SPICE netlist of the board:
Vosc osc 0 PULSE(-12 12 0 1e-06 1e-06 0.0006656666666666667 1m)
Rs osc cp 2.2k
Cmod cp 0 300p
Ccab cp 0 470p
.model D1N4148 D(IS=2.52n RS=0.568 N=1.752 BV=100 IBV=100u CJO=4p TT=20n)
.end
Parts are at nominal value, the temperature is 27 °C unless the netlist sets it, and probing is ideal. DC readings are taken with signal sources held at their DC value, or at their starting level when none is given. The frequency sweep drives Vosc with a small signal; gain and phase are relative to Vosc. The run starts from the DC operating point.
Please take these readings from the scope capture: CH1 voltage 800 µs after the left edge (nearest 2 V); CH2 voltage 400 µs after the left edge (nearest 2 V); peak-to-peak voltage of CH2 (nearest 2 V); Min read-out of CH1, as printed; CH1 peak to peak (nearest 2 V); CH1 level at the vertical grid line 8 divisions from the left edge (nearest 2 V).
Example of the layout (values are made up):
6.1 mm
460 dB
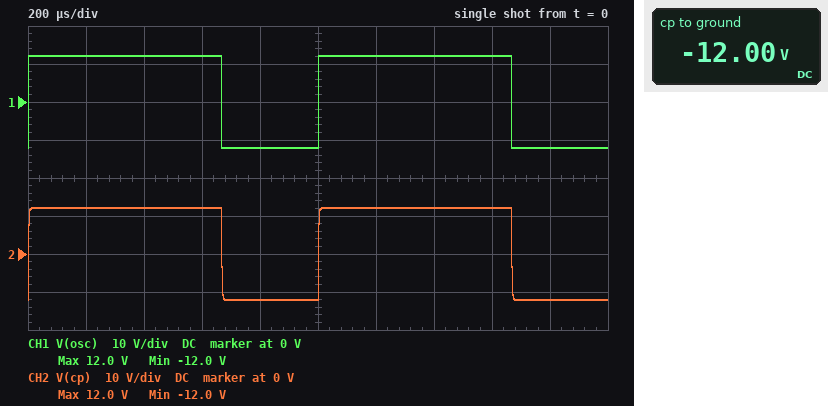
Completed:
-12 V
12 V
24 V
-12.0 V
24 V
12 V
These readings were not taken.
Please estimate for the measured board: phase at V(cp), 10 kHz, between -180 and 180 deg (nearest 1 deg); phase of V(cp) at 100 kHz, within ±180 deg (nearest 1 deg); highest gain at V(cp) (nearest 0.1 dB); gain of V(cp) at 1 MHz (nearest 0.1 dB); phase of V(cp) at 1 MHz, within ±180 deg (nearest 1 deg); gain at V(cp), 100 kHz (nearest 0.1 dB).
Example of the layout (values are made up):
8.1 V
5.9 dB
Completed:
-6 deg
-47 deg
0 dB
-20.6 dB
-85 deg
-3.3 dB
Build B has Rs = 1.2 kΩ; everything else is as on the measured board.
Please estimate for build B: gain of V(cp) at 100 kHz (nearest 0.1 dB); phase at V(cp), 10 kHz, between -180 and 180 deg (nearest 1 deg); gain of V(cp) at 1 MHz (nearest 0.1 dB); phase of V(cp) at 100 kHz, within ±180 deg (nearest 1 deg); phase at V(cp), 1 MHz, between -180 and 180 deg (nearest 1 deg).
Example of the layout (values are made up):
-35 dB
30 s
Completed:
-1.3 dB
-3 deg
-15.4 dB
-30 deg
-80 deg
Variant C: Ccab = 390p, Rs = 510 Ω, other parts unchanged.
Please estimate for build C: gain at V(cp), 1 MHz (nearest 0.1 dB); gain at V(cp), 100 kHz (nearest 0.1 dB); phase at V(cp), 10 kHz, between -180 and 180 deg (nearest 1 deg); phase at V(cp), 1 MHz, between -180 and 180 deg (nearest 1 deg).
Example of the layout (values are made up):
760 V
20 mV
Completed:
-7.7 dB
-0.2 dB
-1 deg
-66 deg
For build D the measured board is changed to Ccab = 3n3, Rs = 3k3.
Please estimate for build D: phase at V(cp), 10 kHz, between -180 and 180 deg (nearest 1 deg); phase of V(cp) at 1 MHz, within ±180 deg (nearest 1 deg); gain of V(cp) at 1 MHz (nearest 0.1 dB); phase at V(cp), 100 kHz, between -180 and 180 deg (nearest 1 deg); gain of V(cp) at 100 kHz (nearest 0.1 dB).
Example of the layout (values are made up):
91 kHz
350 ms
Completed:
-37 deg
-89 deg
-37.5 dB
-82 deg
-17.5 dB
